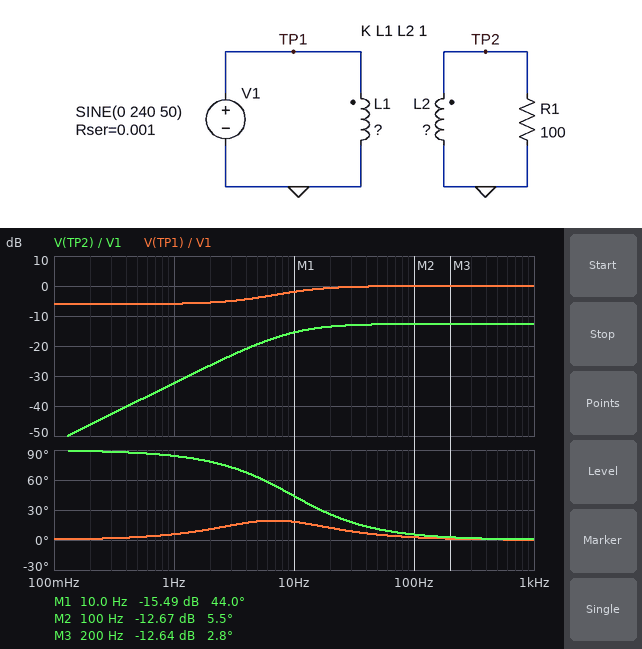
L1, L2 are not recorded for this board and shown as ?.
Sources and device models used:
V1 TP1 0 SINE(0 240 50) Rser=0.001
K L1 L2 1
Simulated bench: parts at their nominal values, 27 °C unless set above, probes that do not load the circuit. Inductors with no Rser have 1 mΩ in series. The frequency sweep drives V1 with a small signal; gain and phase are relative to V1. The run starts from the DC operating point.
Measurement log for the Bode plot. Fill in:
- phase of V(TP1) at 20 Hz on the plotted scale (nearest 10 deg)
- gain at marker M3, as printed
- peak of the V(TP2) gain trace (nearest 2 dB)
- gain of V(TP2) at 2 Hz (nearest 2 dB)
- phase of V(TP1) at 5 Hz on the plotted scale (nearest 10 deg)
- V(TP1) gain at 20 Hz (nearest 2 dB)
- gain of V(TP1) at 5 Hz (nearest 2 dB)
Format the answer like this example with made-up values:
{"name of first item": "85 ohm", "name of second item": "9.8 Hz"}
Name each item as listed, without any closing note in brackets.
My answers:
{"phase of V(TP1) at 20 Hz on the plotted scale": "10 deg", "gain at marker M3, as printed": "-12.64 dB", "peak of the V(TP2) gain trace": "-12 dB", "gain of V(TP2) at 2 Hz": "-26 dB", "phase of V(TP1) at 5 Hz on the plotted scale": "20 deg", "V(TP1) gain at 20 Hz": "0 dB", "gain of V(TP1) at 5 Hz": "-4 dB"}
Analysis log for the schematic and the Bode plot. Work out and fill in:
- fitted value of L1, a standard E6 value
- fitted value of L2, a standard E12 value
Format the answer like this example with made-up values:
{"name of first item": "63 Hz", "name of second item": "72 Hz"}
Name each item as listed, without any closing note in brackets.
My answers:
{"fitted value of L1, a standard E6 value": "33 µH", "fitted value of L2, a standard E12 value": "1.8 µH"}
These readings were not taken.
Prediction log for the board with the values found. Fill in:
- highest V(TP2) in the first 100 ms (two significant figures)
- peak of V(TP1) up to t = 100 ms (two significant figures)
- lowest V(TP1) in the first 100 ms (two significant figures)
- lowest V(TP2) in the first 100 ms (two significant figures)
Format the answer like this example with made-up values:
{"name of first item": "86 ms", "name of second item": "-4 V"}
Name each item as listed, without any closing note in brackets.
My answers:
{"highest V(TP2) in the first 100 ms": "55 V", "peak of V(TP1) up to t = 100 ms": "240 V", "lowest V(TP1) in the first 100 ms": "-250 V", "lowest V(TP2) in the first 100 ms": "-59 V"}
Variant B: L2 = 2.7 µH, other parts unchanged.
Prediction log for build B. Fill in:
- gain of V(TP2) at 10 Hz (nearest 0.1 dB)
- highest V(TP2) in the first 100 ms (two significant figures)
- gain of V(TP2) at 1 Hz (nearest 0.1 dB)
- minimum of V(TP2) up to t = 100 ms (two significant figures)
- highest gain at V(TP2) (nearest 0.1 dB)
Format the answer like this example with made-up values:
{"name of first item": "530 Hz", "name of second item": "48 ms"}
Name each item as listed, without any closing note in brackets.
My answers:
{"gain of V(TP2) at 10 Hz": "-13.7 dB", "highest V(TP2) in the first 100 ms": "67 V", "gain of V(TP2) at 1 Hz": "-30.6 dB", "minimum of V(TP2) up to t = 100 ms": "-73 V", "highest gain at V(TP2)": "-10.9 dB"}
